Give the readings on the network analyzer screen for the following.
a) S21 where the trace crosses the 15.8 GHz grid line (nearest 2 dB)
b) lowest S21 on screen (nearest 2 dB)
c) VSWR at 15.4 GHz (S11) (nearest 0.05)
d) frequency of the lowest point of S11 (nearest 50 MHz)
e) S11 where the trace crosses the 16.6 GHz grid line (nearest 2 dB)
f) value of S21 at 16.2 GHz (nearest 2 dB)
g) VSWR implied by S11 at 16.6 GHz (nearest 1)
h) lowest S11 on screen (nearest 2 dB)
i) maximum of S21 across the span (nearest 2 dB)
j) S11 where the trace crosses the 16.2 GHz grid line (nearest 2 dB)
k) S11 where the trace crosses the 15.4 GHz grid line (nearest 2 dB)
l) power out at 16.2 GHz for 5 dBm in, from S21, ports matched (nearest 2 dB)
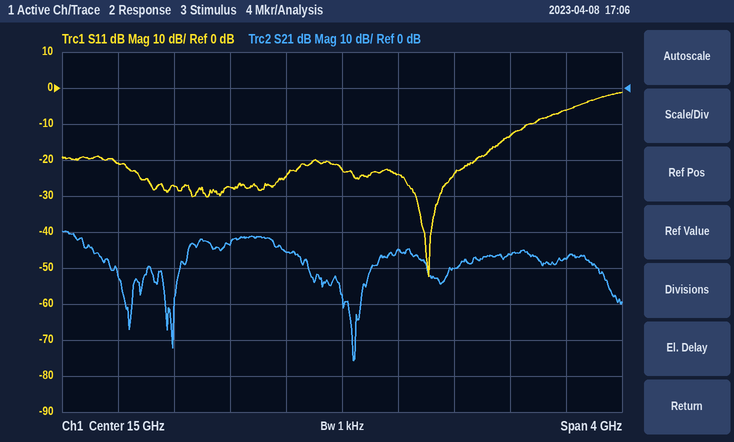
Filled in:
-50 dB
-76 dB
1.15
15.60 GHz
-6 dB
-46 dB
3
-52 dB
-40 dB
-14 dB
-24 dB
-42 dBm
